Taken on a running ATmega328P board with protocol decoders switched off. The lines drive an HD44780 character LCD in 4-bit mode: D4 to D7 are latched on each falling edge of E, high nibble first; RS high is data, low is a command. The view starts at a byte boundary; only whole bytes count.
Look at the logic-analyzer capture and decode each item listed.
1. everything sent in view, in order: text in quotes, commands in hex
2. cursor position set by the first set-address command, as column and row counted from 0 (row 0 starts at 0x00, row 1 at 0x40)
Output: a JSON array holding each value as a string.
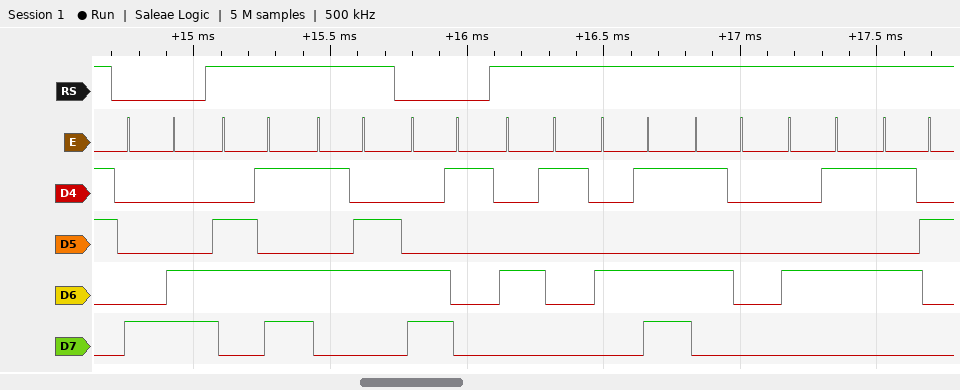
["0x8C \"mV\" 0xC1 \"AMPER\"", "column 12, row 0"]
